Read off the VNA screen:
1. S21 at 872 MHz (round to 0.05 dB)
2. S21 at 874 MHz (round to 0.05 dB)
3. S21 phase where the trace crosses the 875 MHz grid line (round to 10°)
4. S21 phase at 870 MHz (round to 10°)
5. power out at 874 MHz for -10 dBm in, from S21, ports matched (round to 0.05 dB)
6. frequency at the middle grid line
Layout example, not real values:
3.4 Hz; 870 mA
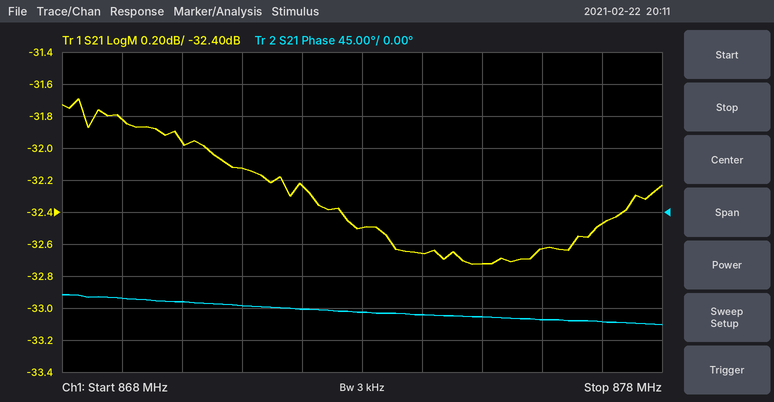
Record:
-32.25 dB; -32.65 dB; -150°; -130°; -42.65 dBm; 873 MHz
